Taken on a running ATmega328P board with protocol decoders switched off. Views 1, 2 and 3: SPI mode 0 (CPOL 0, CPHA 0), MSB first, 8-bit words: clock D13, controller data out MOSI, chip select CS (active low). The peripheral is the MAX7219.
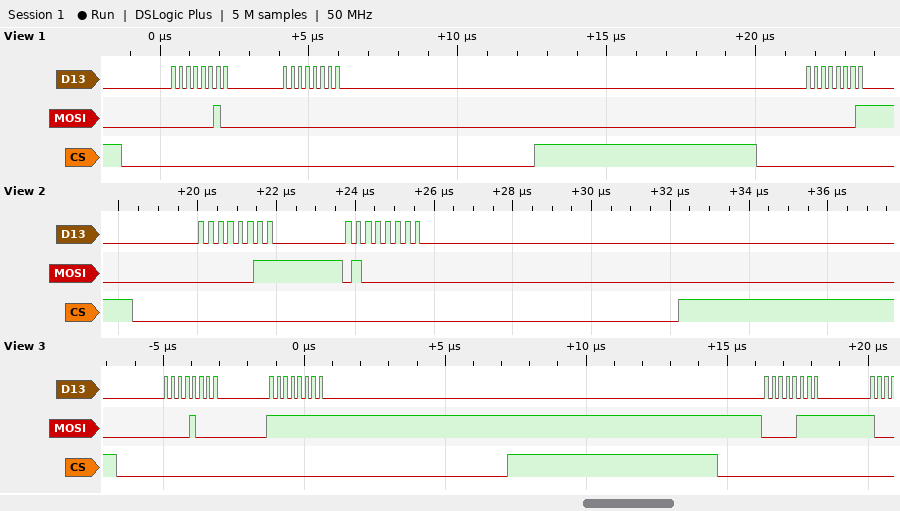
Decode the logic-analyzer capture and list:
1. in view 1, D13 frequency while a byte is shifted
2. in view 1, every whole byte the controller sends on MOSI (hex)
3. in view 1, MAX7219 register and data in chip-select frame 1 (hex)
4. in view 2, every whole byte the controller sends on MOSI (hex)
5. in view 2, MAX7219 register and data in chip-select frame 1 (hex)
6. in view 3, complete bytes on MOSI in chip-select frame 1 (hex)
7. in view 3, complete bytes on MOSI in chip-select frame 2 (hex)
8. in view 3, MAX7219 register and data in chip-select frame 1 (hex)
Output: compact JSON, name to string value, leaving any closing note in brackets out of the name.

{"in view 1, D13 frequency while a byte is shifted": "4 MHz", "in view 1, every whole byte the controller sends on MOSI": "0x02 0x00 0x01", "in view 1, MAX7219 register and data in chip-select frame 1": "register 0x2, data 0x00", "in view 2, every whole byte the controller sends on MOSI": "0x03 0x40", "in view 2, MAX7219 register and data in chip-select frame 1": "register 0x3, data 0x40", "in view 3, complete bytes on MOSI in chip-select frame 1": "08 FF", "in view 3, complete bytes on MOSI in chip-select frame 2": "07", "in view 3, MAX7219 register and data in chip-select frame 1": "register 0x8, data 0xFF"}
